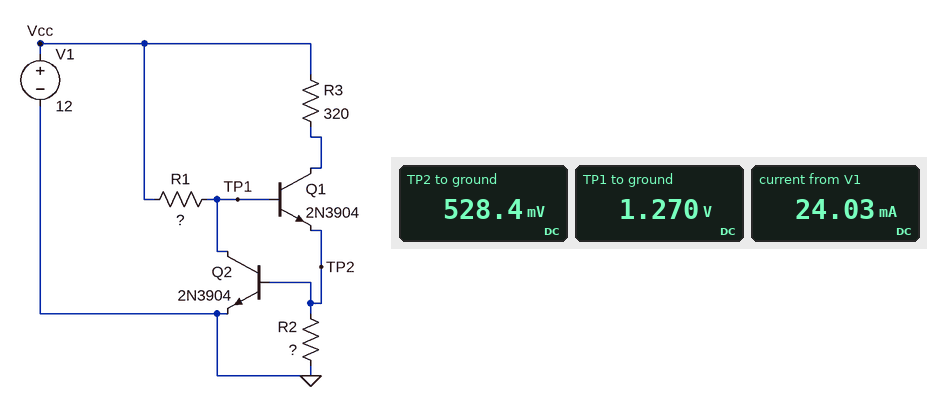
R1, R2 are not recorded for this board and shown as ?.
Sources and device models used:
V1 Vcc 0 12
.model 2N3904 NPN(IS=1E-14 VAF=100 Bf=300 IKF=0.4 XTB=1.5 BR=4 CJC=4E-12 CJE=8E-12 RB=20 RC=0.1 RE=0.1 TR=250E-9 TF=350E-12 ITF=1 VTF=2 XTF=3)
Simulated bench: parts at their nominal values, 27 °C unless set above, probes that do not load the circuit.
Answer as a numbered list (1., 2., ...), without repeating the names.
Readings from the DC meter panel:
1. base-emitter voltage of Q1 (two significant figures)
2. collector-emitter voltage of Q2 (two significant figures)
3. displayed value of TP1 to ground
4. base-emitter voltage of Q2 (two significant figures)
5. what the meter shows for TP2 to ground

1. 740 mV
2. 1.3 V
3. 1.270 V
4. 530 mV
5. 528.4 mV
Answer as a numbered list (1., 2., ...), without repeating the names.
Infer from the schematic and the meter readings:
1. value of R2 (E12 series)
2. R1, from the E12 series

1. 22 Ω
2. 120 kΩ
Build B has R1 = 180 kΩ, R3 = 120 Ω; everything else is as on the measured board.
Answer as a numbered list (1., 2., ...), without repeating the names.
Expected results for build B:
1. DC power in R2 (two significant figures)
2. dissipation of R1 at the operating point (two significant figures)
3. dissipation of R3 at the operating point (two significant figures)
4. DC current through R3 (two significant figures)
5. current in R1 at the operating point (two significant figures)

1. 7.8 mW
2. 650 µW
3. 42 mW
4. 19 mA
5. 60 µA
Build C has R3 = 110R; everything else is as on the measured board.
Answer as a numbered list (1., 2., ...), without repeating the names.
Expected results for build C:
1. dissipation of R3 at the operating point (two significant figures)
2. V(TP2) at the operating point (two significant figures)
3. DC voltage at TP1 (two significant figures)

1. 65 mW
2. 540 mV
3. 1.3 V
